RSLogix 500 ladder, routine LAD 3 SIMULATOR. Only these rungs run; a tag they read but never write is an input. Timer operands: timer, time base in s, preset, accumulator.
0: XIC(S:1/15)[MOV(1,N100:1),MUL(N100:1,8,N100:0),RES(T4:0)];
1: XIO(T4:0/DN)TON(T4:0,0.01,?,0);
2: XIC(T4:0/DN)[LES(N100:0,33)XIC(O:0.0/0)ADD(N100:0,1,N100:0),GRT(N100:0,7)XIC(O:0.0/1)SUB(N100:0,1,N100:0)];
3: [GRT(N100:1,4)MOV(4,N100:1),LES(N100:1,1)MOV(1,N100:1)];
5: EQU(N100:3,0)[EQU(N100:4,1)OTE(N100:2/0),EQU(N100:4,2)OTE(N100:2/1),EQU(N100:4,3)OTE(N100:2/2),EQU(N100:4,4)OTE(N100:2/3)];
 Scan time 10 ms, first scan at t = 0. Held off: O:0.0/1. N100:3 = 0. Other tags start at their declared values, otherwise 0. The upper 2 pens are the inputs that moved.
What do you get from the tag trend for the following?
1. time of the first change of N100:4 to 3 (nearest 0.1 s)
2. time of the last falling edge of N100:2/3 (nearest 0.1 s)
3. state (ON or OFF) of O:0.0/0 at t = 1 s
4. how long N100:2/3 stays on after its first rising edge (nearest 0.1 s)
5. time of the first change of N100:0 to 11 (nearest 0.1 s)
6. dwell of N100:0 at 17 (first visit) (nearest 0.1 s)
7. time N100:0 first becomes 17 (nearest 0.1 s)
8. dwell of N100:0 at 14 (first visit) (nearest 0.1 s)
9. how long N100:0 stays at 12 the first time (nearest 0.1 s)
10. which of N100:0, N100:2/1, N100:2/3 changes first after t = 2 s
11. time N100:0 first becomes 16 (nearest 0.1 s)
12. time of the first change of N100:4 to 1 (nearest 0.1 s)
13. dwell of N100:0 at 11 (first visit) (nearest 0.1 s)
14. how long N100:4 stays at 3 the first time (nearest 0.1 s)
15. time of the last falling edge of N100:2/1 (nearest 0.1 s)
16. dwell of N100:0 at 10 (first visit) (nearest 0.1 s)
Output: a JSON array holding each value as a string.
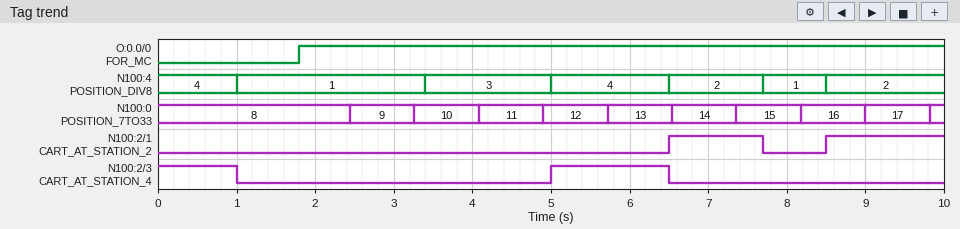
["3.4 s", "6.5 s", "OFF", "1.5 s", "4.1 s", "0.8 s", "9.0 s", "0.8 s", "0.8 s", "N100:0", "8.2 s", "1.0 s", "0.8 s", "1.6 s", "7.7 s", "0.8 s"]
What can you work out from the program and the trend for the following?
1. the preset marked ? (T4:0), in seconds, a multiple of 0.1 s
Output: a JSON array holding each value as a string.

["0.8 s"]
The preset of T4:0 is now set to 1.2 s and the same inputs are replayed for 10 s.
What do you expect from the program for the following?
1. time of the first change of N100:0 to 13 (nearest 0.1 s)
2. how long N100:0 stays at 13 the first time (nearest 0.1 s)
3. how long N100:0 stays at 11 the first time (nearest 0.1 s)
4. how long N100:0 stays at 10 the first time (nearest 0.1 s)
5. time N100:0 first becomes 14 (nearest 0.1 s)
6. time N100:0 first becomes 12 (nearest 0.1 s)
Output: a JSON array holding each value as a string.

["7.3 s", "1.2 s", "1.2 s", "1.2 s", "8.5 s", "6.1 s"]
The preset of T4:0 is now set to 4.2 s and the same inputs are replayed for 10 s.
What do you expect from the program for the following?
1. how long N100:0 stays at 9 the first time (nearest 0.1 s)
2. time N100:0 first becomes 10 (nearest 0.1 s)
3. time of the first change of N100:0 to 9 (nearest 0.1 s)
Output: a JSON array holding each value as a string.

["4.2 s", "8.4 s", "4.2 s"]
